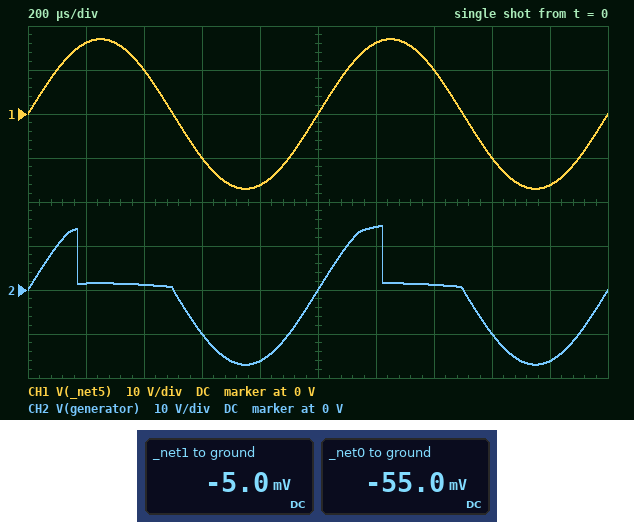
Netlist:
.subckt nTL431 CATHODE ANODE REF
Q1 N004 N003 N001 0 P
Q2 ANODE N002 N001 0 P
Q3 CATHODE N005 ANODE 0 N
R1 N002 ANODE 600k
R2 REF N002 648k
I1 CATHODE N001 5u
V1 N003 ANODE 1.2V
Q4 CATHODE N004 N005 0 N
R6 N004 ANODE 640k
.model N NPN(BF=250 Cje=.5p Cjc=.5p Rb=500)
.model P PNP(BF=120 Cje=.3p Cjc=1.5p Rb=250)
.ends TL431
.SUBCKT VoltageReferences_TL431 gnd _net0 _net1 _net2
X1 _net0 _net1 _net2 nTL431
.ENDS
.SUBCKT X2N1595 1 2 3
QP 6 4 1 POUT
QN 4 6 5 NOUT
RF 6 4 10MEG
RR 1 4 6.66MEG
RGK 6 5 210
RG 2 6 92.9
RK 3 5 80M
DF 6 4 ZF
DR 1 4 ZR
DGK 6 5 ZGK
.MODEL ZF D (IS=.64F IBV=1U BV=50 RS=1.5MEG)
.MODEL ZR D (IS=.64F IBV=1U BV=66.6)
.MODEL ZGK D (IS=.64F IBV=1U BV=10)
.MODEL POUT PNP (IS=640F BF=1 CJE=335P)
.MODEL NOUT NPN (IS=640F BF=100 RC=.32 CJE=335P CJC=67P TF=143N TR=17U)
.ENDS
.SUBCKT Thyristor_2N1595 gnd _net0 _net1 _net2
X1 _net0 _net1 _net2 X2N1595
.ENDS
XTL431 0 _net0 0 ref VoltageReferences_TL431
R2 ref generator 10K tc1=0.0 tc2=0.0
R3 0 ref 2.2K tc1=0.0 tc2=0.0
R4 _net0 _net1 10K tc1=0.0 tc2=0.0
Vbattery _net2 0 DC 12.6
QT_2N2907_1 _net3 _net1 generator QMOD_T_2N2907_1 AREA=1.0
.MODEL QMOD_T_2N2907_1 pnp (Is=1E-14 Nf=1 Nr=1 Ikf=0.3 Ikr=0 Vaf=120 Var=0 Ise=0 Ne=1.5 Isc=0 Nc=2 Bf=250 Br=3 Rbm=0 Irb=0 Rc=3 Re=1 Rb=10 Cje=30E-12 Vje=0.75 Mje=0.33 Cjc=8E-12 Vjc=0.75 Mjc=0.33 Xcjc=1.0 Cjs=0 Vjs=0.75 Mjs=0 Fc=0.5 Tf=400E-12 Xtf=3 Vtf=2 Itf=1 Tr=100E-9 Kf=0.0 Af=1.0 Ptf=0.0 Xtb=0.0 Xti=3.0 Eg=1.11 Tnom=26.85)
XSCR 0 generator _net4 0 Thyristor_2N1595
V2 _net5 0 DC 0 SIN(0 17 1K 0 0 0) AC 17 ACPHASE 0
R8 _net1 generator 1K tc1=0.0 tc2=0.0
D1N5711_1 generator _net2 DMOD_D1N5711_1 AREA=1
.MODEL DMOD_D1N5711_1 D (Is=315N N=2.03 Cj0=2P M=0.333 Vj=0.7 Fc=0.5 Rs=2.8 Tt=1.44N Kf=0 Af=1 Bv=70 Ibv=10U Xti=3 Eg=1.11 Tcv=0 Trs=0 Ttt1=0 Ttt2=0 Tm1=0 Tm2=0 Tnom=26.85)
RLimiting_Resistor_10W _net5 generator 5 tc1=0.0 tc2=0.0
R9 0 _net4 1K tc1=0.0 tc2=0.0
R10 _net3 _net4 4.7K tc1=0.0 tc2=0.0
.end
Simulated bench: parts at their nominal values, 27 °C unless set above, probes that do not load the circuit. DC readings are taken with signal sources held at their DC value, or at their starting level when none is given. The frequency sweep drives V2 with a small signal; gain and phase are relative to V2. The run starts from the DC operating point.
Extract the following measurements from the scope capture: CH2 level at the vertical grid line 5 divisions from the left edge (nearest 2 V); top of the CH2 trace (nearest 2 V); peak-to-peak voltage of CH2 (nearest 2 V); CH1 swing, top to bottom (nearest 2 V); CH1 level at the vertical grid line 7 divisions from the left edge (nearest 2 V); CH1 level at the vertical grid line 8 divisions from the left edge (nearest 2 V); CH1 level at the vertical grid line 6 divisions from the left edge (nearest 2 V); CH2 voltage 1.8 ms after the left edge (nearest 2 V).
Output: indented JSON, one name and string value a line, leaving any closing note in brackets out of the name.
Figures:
{
  "CH2 level at the vertical grid line 5 divisions from the left edge": "0 V",
  "top of the CH2 trace": "14 V",
  "peak-to-peak voltage of CH2": "32 V",
  "CH1 swing, top to bottom": "34 V",
  "CH1 level at the vertical grid line 7 divisions from the left edge": "10 V",
  "CH1 level at the vertical grid line 8 divisions from the left edge": "-10 V",
  "CH1 level at the vertical grid line 6 divisions from the left edge": "16 V",
  "CH2 voltage 1.8 ms after the left edge": "-16 V"
}
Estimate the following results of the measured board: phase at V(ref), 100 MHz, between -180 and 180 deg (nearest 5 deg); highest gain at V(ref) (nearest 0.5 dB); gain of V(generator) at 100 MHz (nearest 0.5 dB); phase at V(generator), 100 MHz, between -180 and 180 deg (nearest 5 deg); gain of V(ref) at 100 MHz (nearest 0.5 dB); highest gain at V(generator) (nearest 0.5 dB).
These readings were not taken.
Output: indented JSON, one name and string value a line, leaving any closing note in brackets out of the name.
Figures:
{
  "phase at V(ref), 100 MHz, between -180 and 180 deg": "-10 deg",
  "highest gain at V(ref)": "-15.0 dB",
  "gain of V(generator) at 100 MHz": "0 dB",
  "phase at V(generator), 100 MHz, between -180 and 180 deg": "-10 deg",
  "gain of V(ref) at 100 MHz": "-15.0 dB",
  "highest gain at V(generator)": "0 dB"
}
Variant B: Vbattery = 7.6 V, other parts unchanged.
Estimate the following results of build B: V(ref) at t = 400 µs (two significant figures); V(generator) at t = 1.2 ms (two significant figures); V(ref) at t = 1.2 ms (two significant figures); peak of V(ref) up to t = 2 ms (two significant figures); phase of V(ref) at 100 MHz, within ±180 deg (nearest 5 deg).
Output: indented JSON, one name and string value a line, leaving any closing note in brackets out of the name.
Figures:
{
  "V(ref) at t = 400 µs": "1.6 V",
  "V(generator) at t = 1.2 ms": "11 V",
  "V(ref) at t = 1.2 ms": "2.0 V",
  "peak of V(ref) up to t = 2 ms": "2.1 V",
  "phase of V(ref) at 100 MHz, within ±180 deg": "-10 deg"
}
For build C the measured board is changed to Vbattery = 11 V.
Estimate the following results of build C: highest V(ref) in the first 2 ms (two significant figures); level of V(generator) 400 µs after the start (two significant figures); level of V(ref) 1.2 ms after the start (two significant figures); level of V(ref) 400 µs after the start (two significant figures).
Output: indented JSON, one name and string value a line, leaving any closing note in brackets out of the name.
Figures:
{
  "highest V(ref) in the first 2 ms": "2.5 V",
  "level of V(generator) 400 µs after the start": "10 V",
  "level of V(ref) 1.2 ms after the start": "2.4 V",
  "level of V(ref) 400 µs after the start": "1.8 V"
}
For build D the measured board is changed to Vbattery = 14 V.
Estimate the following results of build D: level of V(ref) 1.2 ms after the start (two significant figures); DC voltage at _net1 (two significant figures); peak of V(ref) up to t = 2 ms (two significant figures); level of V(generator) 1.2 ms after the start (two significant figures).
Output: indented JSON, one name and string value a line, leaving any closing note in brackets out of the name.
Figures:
{
  "level of V(ref) 1.2 ms after the start": "270 mV",
  "DC voltage at _net1": "-5.0 mV",
  "peak of V(ref) up to t = 2 ms": "2.7 V",
  "level of V(generator) 1.2 ms after the start": "1.5 V"
}
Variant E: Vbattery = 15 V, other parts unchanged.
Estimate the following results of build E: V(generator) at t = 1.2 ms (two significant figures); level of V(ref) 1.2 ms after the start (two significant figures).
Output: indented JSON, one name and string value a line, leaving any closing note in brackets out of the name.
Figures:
{
  "V(generator) at t = 1.2 ms": "1.5 V",
  "level of V(ref) 1.2 ms after the start": "270 mV"
}
